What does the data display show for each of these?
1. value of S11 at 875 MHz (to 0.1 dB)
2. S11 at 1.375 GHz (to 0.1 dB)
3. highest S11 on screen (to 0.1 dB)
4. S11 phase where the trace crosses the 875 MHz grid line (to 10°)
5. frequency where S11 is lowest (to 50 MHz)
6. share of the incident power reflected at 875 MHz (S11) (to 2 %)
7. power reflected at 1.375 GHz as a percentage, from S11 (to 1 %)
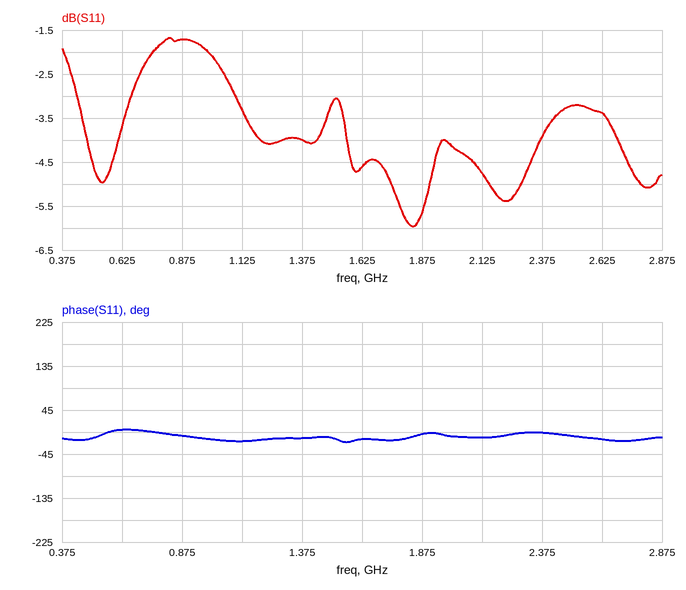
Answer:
-1.7 dB
-4.0 dB
-1.7 dB
-10°
1.85 GHz
68 %
40 %
